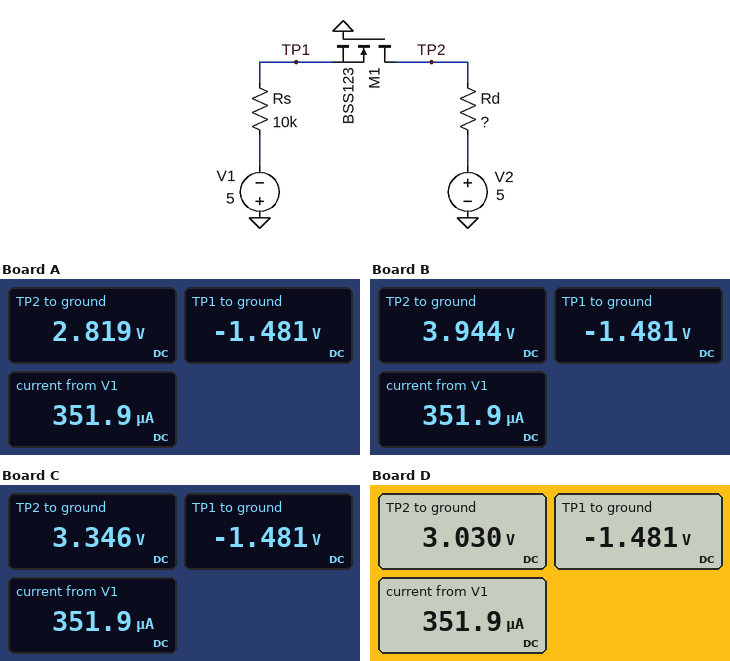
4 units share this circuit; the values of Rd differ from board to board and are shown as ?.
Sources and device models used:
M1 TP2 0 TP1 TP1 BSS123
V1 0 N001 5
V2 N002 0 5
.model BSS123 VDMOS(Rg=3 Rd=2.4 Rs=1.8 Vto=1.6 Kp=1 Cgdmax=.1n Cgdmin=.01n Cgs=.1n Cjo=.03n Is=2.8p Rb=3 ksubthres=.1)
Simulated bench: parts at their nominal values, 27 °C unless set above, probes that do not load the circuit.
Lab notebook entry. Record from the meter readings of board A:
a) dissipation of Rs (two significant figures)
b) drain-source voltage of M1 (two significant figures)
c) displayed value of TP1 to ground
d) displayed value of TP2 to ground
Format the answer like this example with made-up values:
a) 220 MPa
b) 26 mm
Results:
a) 1.2 mW
b) 4.3 V
c) -1.481 V
d) 2.819 V
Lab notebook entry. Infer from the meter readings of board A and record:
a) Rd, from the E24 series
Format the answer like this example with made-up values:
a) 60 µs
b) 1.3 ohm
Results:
a) 6.2 kΩ
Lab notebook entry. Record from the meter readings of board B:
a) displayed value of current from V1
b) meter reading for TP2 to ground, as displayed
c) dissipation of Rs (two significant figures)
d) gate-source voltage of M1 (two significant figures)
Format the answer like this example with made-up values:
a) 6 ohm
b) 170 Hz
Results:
a) 351.9 µA
b) 3.944 V
c) 1.2 mW
d) 1.5 V
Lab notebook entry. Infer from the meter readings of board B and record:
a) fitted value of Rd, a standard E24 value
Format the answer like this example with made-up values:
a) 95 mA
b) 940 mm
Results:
a) 3 kΩ
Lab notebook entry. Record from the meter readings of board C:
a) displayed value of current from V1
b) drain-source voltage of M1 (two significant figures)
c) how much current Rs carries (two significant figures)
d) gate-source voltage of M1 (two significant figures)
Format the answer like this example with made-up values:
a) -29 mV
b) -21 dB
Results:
a) 351.9 µA
b) 4.8 V
c) 350 µA
d) 1.5 V
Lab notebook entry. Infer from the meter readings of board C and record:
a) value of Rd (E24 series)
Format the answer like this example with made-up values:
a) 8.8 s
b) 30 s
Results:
a) 4.7 kΩ
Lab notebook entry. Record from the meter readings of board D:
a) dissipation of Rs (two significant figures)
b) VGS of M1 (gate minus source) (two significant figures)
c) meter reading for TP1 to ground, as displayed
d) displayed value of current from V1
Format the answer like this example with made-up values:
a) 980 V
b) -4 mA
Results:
a) 1.2 mW
b) 1.5 V
c) -1.481 V
d) 351.9 µA
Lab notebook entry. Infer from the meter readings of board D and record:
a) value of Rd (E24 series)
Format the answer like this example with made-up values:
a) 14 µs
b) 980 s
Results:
a) 5.6 kΩ
